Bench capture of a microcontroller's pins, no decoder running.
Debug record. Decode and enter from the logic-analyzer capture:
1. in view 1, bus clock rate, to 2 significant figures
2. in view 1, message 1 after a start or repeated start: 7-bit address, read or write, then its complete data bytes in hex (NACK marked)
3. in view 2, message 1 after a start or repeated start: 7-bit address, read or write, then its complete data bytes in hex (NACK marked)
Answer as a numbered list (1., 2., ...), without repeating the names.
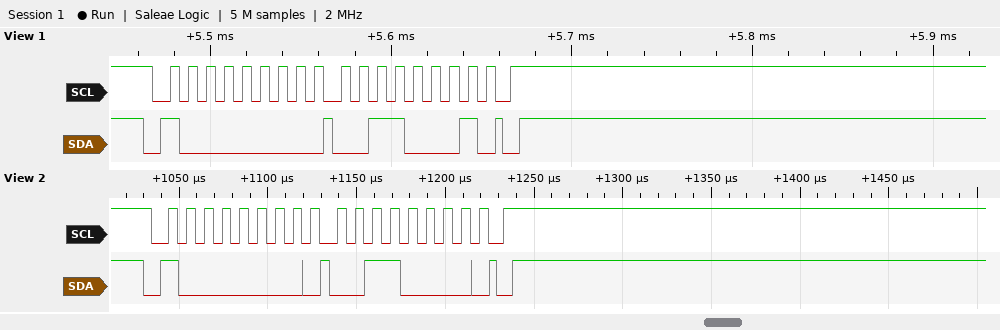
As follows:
1. 100 kHz
2. 0x40 write: 31
3. 0x40 write: 30
